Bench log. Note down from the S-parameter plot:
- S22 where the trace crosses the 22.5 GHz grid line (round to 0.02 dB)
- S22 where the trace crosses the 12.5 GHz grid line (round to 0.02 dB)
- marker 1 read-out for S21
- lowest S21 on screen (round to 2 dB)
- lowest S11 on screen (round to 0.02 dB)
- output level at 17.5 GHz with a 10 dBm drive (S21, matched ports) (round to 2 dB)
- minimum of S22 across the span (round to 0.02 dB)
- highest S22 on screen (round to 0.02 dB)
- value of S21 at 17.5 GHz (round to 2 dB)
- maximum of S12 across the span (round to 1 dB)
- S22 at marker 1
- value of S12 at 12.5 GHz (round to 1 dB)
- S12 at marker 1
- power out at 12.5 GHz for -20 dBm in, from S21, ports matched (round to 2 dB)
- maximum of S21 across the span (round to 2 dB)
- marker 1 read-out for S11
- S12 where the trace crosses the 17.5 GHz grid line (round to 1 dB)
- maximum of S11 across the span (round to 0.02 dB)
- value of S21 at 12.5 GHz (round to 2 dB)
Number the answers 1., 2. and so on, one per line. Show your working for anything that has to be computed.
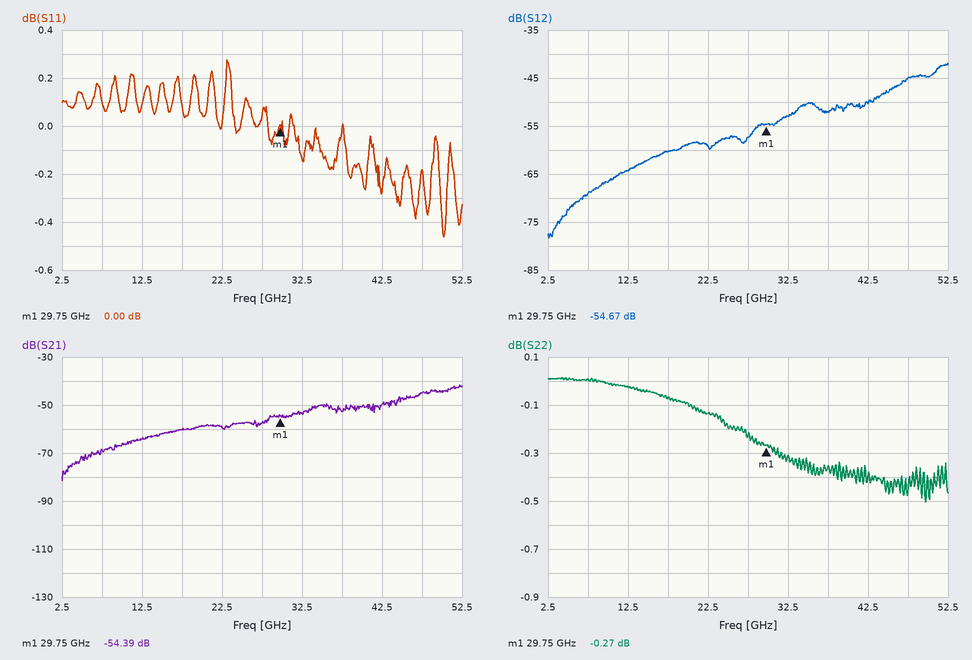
1. -0.14 dB
2. -0.02 dB
3. -54.39 dB
4. -82 dB
5. -0.46 dB
6. 10 dBm + (-60 dB) = -50 dBm
7. -0.50 dB
8. 0.02 dB
9. -60 dB
10. -42 dB
11. -0.27 dB
12. -64 dB
13. -54.67 dB
14. -20 dBm + (-64 dB) = -84 dBm
15. -42 dB
16. 0.00 dB
17. -60 dB
18. 0.28 dB
19. -64 dB
